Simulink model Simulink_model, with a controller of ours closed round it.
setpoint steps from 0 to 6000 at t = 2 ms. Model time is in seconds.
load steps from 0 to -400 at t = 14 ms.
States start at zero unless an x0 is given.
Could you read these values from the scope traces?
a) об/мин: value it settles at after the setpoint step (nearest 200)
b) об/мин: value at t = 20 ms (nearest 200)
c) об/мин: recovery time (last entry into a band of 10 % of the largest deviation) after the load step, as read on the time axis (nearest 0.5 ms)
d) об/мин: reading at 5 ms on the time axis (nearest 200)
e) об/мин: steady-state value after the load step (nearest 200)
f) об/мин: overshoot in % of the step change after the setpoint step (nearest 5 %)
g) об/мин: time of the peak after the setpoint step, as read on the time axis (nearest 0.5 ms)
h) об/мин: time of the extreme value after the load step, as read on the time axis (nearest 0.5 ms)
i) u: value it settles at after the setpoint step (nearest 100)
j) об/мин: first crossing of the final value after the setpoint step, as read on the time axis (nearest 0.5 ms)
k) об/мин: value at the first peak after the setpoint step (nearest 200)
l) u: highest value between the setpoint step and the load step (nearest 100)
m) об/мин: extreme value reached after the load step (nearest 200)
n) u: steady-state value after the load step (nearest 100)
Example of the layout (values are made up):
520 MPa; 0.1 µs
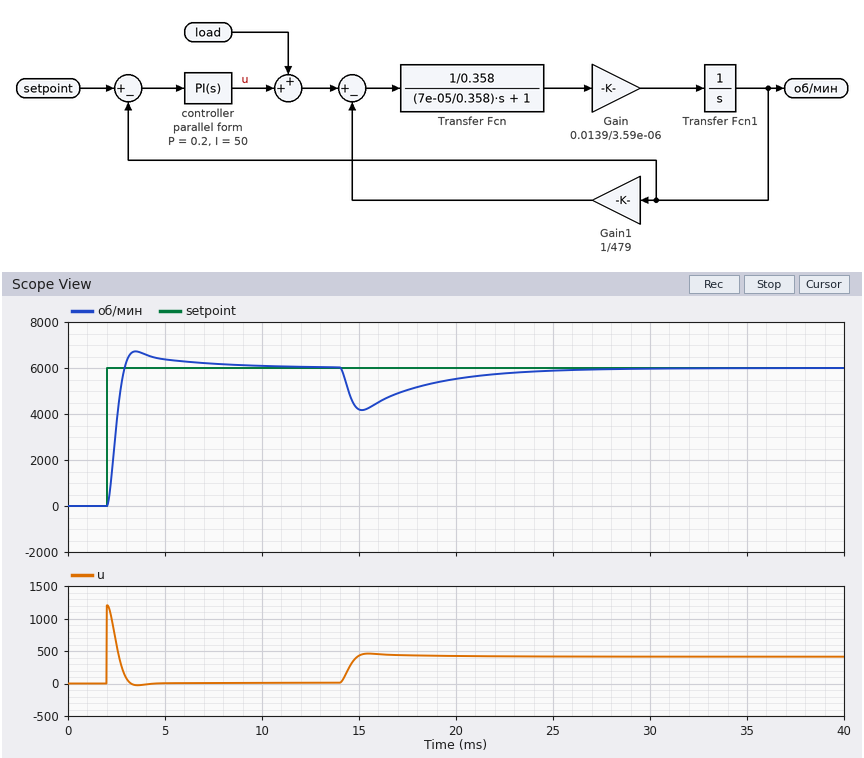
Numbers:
6000; 5600; 23.5 ms; 6400; 6000; 10 %; 3.5 ms; 15.0 ms; 0; 3.0 ms; 6800; 1200; 4200; 400
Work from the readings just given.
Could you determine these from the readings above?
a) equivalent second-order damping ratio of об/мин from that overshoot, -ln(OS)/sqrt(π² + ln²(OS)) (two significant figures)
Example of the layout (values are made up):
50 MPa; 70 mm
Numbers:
0.59
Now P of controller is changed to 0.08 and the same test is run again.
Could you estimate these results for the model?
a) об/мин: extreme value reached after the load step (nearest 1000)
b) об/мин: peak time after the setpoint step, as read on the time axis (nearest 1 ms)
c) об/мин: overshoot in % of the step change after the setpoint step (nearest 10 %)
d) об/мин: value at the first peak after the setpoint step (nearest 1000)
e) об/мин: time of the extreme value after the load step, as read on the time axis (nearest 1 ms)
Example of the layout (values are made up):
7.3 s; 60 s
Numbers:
3000; 5 ms; 30 %; 8000; 16 ms
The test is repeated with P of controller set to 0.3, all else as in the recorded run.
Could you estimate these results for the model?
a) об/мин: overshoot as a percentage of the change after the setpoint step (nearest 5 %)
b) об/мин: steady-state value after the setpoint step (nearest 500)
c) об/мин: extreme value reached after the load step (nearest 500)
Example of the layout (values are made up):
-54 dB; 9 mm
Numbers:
15 %; 6000; 4500
